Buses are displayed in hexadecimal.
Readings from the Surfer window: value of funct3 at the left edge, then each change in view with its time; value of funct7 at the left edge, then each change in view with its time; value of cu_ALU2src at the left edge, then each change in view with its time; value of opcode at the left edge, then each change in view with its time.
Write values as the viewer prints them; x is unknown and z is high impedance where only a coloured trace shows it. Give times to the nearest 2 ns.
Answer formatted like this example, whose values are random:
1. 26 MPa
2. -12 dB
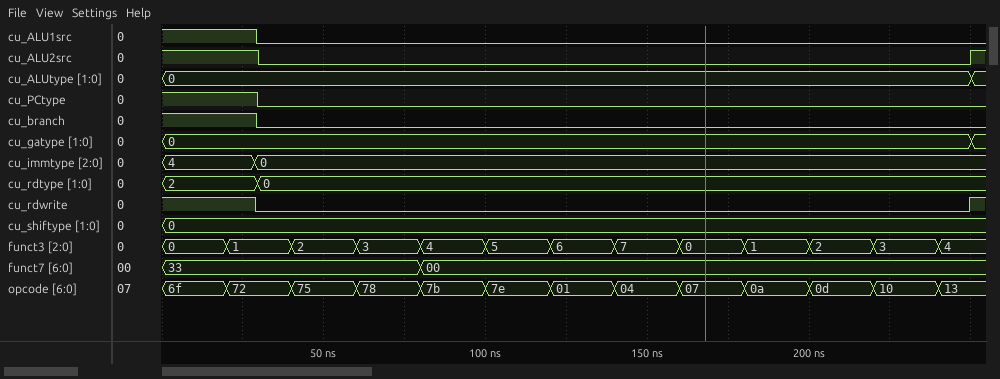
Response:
1. 0, 1 at 20 ns, 2 at 40 ns, 3 at 60 ns, 4 at 80 ns, 5 at 100 ns, 6 at 120 ns, 7 at 140 ns, 0 at 160 ns, 1 at 180 ns, 2 at 200 ns, 3 at 220 ns, 4 at 240 ns
2. 33, 00 at 80 ns
3. 1, 0 at 30 ns, 1 at 250 ns
4. 6f, 72 at 20 ns, 75 at 40 ns, 78 at 60 ns, 7b at 80 ns, 7e at 100 ns, 01 at 120 ns, 04 at 140 ns, 07 at 160 ns, 0a at 180 ns, 0d at 200 ns, 10 at 220 ns, 13 at 240 ns
